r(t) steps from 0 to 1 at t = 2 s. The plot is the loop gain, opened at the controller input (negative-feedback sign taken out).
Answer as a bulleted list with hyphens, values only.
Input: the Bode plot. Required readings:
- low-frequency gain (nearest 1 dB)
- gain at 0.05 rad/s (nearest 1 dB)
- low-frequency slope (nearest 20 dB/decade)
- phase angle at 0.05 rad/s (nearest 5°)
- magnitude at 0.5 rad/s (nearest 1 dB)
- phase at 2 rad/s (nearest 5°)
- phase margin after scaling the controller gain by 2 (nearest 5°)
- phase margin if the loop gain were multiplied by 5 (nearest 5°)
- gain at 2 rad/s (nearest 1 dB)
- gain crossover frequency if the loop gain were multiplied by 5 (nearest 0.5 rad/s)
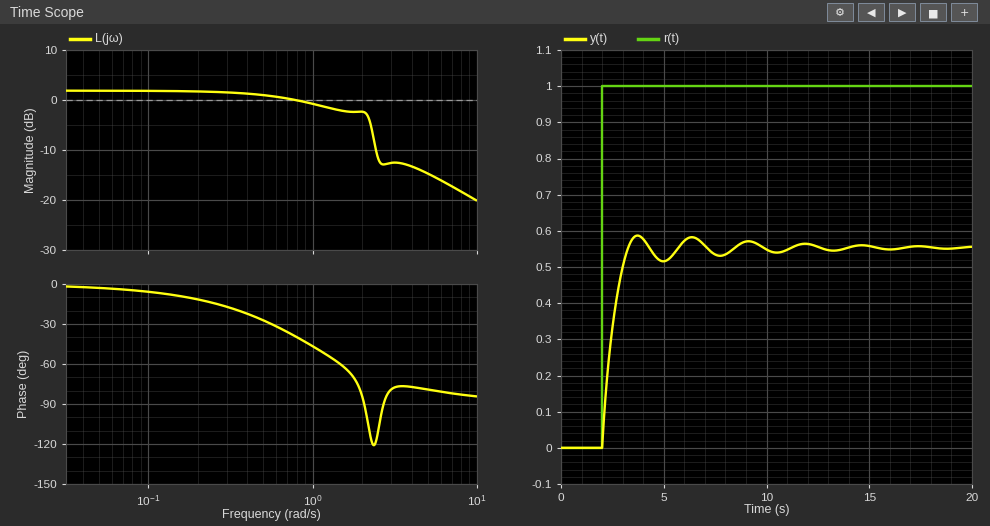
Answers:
- 2 dB
- 2 dB
- 0 dB/decade
- -5°
- 1 dB
- -85°
- 60°
- 100°
- -2 dB
- 4.5 rad/s
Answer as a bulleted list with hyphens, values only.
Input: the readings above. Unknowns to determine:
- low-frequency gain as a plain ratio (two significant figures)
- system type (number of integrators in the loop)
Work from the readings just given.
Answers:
- 1.3
- 0
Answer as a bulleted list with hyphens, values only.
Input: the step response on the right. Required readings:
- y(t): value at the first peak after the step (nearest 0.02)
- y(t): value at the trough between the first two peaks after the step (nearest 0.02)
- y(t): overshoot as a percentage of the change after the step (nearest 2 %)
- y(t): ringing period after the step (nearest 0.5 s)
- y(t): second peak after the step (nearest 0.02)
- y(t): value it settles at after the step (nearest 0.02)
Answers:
- 0.58
- 0.52
- 6 %
- 2.5 s
- 0.58
- 0.56
